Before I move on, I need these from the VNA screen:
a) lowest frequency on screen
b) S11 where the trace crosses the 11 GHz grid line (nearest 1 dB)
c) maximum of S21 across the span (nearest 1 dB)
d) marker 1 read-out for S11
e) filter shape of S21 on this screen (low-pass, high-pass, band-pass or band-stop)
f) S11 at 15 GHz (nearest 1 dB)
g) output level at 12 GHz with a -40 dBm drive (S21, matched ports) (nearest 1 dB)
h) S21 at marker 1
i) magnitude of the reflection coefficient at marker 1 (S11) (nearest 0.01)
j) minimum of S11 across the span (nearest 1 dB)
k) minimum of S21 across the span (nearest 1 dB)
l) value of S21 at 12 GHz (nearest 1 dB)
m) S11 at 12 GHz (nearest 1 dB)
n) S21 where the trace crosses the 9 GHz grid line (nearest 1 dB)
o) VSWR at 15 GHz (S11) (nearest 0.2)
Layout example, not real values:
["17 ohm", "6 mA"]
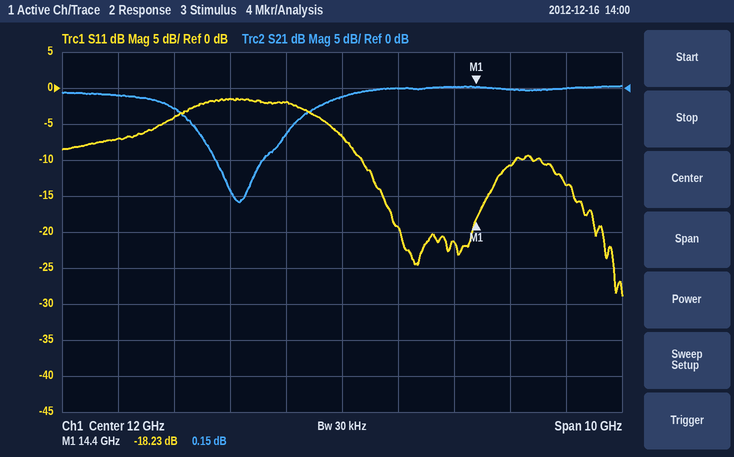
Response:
["7 GHz", "-2 dB", "0 dB", "-18.23 dB", "band-stop", "-11 dB", "-41 dBm", "0.15 dB", "0.12", "-29 dB", "-16 dB", "-1 dB", "-7 dB", "-3 dB", "1.8"]
